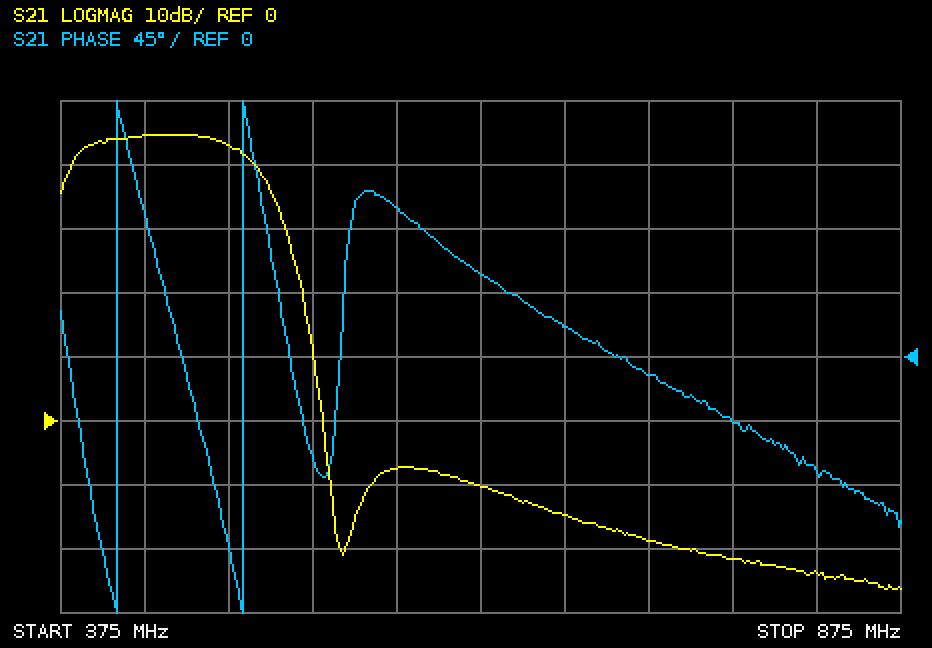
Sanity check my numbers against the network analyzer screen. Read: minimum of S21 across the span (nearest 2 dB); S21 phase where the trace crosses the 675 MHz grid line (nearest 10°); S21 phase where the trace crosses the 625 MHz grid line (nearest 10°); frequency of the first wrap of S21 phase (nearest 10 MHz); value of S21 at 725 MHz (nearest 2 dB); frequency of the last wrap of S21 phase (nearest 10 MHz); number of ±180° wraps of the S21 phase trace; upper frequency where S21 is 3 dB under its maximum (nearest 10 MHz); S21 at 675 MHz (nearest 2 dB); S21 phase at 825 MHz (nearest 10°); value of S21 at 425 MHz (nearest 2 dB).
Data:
-26 dB
20°
60°
410 MHz
-18 dB
480 MHz
2
480 MHz
-14 dB
-80°
44 dB
